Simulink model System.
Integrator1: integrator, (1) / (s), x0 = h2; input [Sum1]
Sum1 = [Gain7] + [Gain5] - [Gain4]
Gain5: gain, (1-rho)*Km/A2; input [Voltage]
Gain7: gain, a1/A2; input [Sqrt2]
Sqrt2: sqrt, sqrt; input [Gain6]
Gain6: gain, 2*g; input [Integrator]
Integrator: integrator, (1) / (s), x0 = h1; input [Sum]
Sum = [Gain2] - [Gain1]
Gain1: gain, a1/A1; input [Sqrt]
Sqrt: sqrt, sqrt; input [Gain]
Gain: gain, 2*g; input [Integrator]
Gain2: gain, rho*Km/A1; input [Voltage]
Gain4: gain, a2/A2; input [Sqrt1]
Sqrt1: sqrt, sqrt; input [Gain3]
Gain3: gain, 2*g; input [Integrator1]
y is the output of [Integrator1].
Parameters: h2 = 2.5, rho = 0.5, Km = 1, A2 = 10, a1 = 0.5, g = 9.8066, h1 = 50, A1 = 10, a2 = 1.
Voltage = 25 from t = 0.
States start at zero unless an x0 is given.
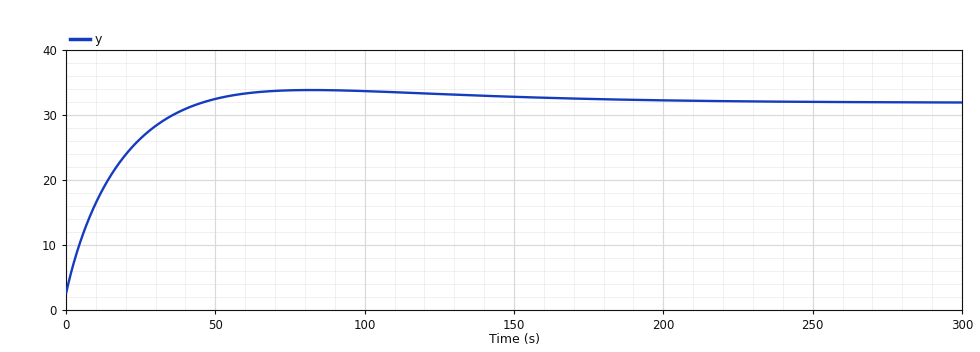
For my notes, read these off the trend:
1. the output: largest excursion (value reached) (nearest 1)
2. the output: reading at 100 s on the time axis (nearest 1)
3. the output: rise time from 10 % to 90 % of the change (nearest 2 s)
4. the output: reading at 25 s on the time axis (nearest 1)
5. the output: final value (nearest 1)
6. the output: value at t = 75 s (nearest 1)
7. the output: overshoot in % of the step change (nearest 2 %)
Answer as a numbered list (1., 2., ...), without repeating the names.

1. 34
2. 34
3. 30 s
4. 26
5. 32
6. 34
7. 6 %
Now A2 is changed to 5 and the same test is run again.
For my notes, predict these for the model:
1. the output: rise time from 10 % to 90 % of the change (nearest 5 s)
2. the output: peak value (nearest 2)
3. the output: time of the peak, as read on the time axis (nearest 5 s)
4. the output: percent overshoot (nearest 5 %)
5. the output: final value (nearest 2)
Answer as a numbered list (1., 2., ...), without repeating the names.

1. 15 s
2. 36
3. 45 s
4. 15 %
5. 32
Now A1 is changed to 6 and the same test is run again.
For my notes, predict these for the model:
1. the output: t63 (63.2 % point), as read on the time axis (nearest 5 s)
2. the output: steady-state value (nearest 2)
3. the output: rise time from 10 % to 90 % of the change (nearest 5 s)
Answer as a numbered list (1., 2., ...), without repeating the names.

1. 15 s
2. 32
3. 35 s
